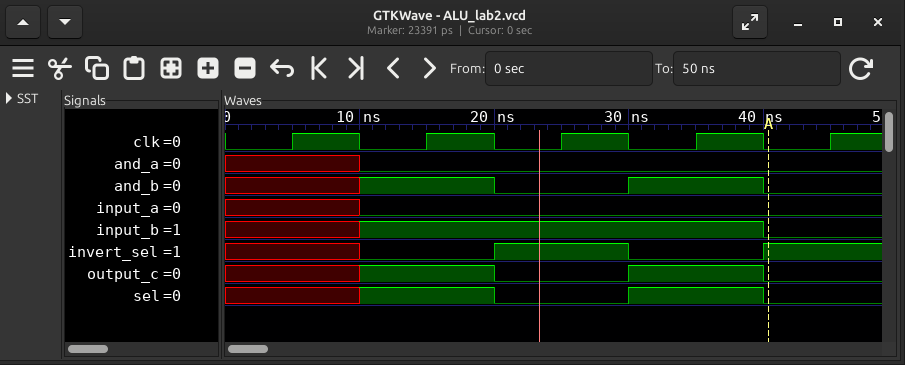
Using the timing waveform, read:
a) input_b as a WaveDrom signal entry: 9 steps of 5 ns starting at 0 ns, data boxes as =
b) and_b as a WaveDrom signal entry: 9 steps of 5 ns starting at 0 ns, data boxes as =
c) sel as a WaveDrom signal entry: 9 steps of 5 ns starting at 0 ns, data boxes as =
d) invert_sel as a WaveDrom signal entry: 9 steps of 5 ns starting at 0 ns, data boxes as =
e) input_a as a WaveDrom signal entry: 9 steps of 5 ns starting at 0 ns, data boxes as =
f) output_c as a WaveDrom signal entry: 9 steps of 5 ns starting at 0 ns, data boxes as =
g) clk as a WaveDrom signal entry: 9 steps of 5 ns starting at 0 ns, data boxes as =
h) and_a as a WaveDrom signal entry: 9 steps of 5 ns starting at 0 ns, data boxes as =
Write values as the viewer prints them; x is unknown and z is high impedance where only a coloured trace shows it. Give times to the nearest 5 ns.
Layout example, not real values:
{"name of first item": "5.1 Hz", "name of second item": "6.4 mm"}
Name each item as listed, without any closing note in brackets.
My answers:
{"input_b as a WaveDrom signal entry: 9 steps of 5 ns starting at 0 ns, data boxes as =": "{name: 'input_b', wave: 'x.1.....0'}", "and_b as a WaveDrom signal entry: 9 steps of 5 ns starting at 0 ns, data boxes as =": "{name: 'and_b', wave: 'x.1.0.1.0'}", "sel as a WaveDrom signal entry: 9 steps of 5 ns starting at 0 ns, data boxes as =": "{name: 'sel', wave: 'x.1.0.1.0'}", "invert_sel as a WaveDrom signal entry: 9 steps of 5 ns starting at 0 ns, data boxes as =": "{name: 'invert_sel', wave: 'x.0.1.0.1'}", "input_a as a WaveDrom signal entry: 9 steps of 5 ns starting at 0 ns, data boxes as =": "{name: 'input_a', wave: 'x.0......'}", "output_c as a WaveDrom signal entry: 9 steps of 5 ns starting at 0 ns, data boxes as =": "{name: 'output_c', wave: 'x.1.0.1.0'}", "clk as a WaveDrom signal entry: 9 steps of 5 ns starting at 0 ns, data boxes as =": "{name: 'clk', wave: '010101010'}", "and_a as a WaveDrom signal entry: 9 steps of 5 ns starting at 0 ns, data boxes as =": "{name: 'and_a', wave: 'x.0......'}"}
